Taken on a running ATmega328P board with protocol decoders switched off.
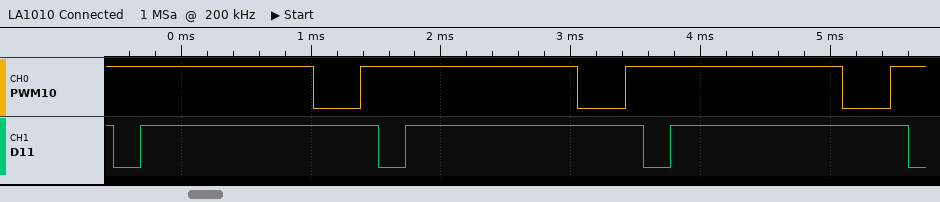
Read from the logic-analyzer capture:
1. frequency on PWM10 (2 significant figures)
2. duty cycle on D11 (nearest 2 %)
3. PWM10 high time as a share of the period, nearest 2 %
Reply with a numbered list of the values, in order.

1. 490 Hz
2. 90 %
3. 82 %
